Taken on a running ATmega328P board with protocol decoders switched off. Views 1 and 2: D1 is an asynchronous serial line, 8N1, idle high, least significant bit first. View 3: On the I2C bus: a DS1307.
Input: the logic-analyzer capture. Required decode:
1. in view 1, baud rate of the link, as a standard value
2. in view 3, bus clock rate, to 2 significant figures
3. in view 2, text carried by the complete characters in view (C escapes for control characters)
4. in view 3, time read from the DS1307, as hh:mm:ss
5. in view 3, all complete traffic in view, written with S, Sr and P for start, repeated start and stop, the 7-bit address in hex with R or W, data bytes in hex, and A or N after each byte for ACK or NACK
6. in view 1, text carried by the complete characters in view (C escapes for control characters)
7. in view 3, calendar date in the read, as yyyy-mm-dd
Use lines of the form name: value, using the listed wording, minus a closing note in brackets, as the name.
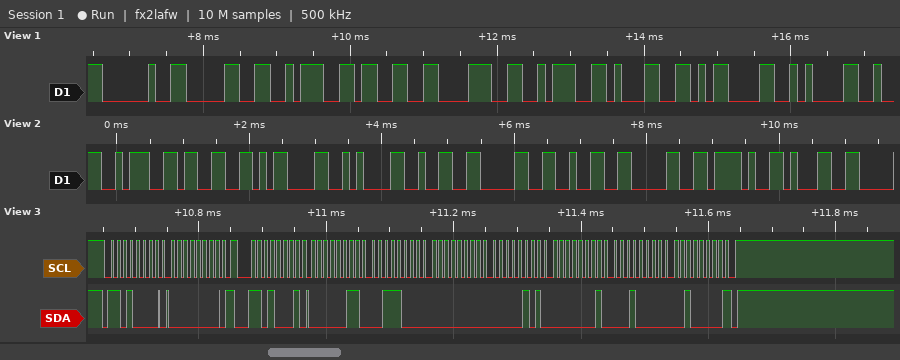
in view 1, baud rate of the link, as a standard value: 9600 baud
in view 3, bus clock rate, to 2 significant figures: 100 kHz
in view 2, text carried by the complete characters in view: ":3\r\n2020/1"
in view 3, time read from the DS1307, as hh:mm:ss: 00:38:03
in view 3, all complete traffic in view, written with S, Sr and P for start, repeated start and stop, the 7-bit address in hex with R or W, data bytes in hex, and A or N after each byte for ACK or NACK: S 68W A 00 A Sr 68R A 03 A 38 A 00 A 05 A 01 A 10 A 20 N P
in view 1, text carried by the complete characters in view: " 0:38:1\r\n"
in view 3, calendar date in the read, as yyyy-mm-dd: 2020-10-01
